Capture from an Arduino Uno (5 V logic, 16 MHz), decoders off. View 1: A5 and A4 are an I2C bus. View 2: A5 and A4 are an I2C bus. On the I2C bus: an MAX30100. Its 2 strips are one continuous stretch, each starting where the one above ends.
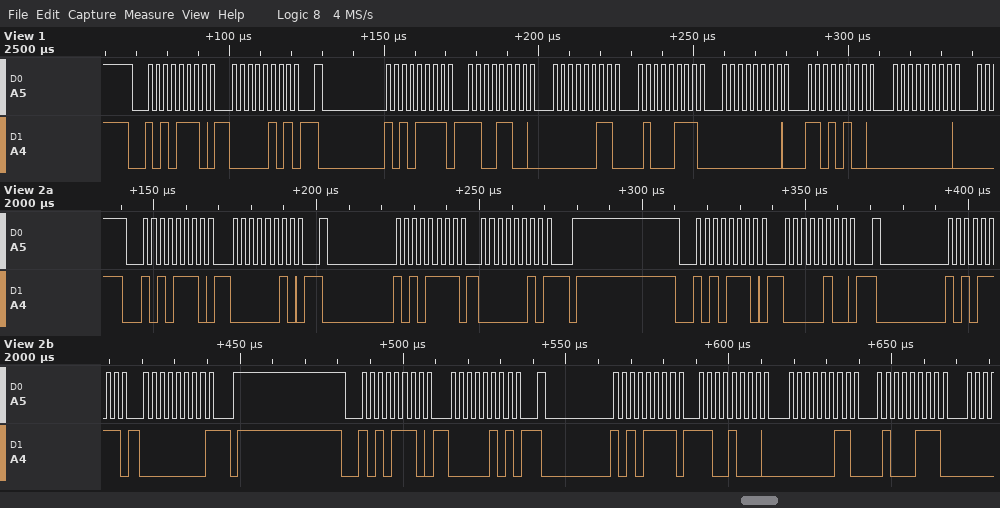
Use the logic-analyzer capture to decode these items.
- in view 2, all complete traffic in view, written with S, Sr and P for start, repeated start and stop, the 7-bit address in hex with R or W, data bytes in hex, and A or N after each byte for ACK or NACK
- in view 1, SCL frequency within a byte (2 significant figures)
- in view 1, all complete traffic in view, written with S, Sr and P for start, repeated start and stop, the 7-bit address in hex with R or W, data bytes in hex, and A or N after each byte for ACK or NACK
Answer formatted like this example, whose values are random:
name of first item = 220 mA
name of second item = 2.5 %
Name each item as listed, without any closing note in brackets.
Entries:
in view 2, all complete traffic in view, written with S, Sr and P for start, repeated start and stop, the 7-bit address in hex with R or W, data bytes in hex, and A or N after each byte for ACK or NACK = S 57W A 02 A Sr 57R A 02 N P S 57W A 04 A Sr 57R A 00 N P S 57W A 05 A Sr 57R A C8 A 03 A 47 A
in view 1, SCL frequency within a byte = 400 kHz
in view 1, all complete traffic in view, written with S, Sr and P for start, repeated start and stop, the 7-bit address in hex with R or W, data bytes in hex, and A or N after each byte for ACK or NACK = S 57W A 05 A Sr 57R A CC A 03 A 47 A 00 A D4 A 00 A
